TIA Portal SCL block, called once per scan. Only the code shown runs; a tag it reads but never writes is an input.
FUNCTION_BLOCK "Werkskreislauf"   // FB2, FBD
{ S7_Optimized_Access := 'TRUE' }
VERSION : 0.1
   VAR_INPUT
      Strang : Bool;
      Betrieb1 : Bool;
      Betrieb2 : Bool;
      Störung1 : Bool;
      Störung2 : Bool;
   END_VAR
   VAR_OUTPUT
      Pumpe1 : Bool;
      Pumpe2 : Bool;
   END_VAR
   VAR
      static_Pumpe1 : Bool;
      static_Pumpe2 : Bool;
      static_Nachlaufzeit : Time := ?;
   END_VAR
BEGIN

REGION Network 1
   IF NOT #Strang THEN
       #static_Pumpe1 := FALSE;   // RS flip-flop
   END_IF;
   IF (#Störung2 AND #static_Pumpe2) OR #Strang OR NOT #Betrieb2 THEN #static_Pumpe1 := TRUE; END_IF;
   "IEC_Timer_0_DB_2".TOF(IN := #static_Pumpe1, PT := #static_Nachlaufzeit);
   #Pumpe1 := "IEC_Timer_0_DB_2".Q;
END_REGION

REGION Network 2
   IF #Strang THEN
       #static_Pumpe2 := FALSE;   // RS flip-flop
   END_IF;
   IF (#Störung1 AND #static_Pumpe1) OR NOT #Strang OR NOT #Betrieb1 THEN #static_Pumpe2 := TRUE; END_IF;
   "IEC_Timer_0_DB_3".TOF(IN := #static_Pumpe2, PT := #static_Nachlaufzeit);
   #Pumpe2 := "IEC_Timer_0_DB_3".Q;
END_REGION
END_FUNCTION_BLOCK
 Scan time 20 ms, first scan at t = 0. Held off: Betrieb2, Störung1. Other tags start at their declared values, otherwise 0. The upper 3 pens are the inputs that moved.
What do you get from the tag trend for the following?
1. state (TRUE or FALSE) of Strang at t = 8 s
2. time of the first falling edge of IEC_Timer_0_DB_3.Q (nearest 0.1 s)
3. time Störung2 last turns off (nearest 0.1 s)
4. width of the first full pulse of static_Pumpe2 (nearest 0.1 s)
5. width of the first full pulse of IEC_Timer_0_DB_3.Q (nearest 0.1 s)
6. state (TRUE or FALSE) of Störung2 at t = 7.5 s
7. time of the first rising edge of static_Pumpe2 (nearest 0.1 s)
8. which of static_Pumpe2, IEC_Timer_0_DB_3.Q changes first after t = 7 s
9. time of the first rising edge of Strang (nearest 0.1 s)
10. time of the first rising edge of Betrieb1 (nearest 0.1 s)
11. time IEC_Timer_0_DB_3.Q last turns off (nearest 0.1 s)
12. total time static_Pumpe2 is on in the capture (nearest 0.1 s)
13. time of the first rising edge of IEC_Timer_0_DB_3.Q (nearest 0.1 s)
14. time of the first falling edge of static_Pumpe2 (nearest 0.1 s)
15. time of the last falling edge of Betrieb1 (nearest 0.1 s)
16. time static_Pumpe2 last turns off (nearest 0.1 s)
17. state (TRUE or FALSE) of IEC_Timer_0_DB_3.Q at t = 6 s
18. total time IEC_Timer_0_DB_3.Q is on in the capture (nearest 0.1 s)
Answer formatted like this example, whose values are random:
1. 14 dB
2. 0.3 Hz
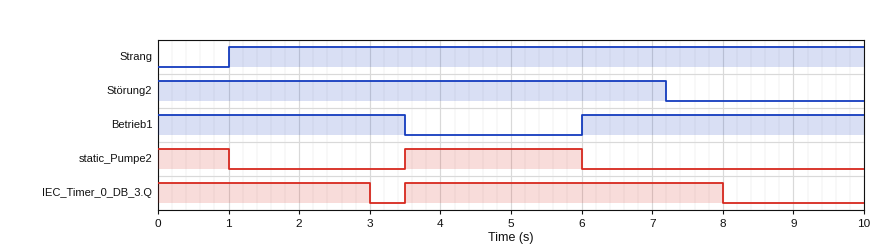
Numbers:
1. TRUE
2. 3.0 s
3. 7.2 s
4. 2.5 s
5. 4.5 s
6. FALSE
7. 3.5 s
8. IEC_Timer_0_DB_3.Q
9. 1.0 s
10. 6.0 s
11. 8.0 s
12. 3.5 s
13. 3.5 s
14. 1.0 s
15. 3.5 s
16. 6.0 s
17. TRUE
18. 7.5 s
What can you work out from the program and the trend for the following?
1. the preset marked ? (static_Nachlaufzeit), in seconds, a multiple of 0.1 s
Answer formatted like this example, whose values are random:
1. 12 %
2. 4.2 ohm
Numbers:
1. 2.0 s
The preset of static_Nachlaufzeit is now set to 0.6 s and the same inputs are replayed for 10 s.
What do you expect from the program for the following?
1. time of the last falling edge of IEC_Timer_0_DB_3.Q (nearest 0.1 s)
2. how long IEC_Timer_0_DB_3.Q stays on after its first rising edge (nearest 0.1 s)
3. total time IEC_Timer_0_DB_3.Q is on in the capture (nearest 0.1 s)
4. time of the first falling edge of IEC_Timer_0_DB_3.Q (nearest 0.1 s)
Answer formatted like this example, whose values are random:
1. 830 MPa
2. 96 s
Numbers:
1. 6.6 s
2. 3.1 s
3. 4.7 s
4. 1.6 s
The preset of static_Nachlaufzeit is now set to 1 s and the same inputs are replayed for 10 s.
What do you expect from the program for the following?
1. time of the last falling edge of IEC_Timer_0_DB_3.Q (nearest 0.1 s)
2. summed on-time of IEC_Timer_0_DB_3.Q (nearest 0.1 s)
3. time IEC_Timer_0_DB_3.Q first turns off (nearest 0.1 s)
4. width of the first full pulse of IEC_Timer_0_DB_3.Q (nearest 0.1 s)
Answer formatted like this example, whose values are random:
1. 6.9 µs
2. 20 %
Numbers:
1. 7.0 s
2. 5.5 s
3. 2.0 s
4. 3.5 s
